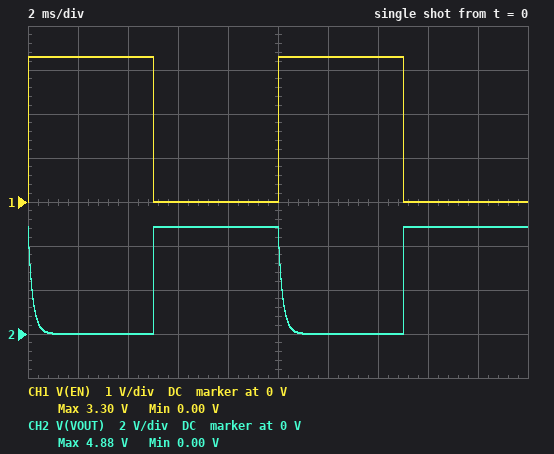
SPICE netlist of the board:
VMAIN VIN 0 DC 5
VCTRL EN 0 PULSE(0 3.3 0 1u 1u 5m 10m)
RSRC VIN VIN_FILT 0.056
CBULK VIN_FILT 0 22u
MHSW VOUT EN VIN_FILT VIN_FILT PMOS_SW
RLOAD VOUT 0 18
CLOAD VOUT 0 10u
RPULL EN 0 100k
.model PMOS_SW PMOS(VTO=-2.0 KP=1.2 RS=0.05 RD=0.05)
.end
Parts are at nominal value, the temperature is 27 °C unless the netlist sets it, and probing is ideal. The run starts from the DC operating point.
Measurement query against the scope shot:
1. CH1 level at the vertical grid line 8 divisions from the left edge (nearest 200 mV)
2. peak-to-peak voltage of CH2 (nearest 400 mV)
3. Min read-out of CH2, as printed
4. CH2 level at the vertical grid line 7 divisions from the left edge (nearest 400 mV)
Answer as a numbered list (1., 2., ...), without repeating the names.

1. 0 V
2. 4.8 V
3. 0.00 V
4. 0 V
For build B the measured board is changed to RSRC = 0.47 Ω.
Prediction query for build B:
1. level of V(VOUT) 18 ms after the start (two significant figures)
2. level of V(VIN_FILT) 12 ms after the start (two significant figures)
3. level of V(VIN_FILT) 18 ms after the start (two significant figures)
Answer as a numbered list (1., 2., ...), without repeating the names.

1. 4.8 V
2. 5.0 V
3. 4.9 V
